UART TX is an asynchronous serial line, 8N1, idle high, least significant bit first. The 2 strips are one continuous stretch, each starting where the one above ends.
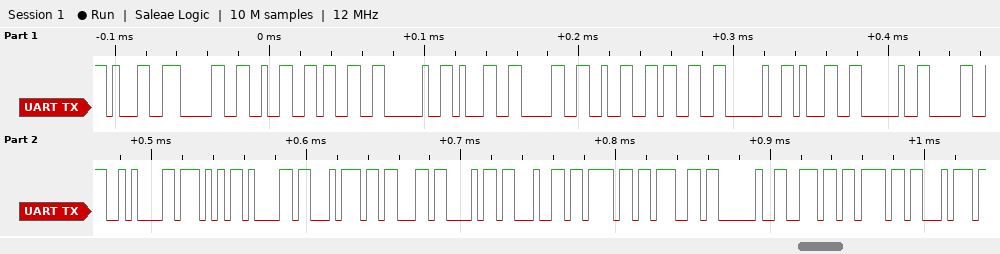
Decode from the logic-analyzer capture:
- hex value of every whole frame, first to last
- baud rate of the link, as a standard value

31 30 32 33 20 31 30 32 33 20 31 20 30 0A 57 61 74 63 68 64 6F 67 20 6E 6F 74
250000 baud
